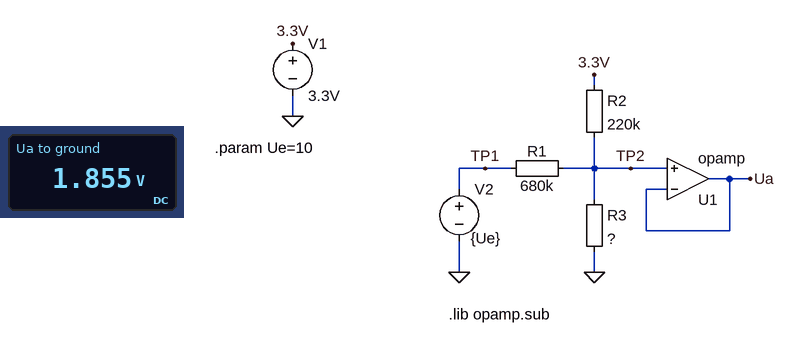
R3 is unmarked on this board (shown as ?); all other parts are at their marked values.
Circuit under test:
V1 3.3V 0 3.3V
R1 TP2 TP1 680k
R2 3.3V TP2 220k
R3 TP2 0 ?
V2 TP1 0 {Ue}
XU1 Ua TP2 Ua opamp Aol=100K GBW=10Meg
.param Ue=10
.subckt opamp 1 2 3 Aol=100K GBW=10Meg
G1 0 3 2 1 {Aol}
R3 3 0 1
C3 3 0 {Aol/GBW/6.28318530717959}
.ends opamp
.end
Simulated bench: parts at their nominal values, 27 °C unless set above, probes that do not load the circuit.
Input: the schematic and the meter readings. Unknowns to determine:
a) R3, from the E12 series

100 kΩ
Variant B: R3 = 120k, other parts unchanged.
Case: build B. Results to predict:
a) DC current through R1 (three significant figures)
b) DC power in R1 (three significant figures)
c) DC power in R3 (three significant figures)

11.7 µA
92.5 µW
35.7 µW
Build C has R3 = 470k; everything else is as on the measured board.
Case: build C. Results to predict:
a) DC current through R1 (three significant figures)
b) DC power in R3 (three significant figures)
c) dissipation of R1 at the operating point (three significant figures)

9.34 µA
28.3 µW
59.3 µW
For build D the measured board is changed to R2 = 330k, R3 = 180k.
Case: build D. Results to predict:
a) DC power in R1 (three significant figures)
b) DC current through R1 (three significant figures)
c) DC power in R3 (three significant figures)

83.7 µW
11.1 µA
33.5 µW
